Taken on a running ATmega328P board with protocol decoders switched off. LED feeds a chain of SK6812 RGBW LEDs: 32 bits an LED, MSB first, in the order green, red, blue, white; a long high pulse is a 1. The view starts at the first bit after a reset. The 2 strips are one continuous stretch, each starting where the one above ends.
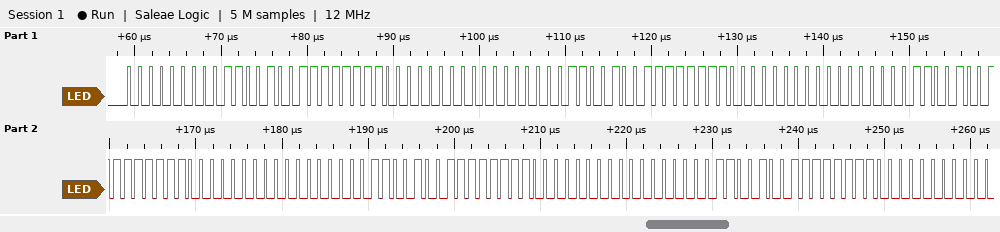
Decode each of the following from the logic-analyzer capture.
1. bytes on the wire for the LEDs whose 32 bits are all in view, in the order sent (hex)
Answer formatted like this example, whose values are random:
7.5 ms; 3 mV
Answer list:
00 64 FF 00 00 64 FF 00 00 64 FF 00 00 64 FF 00 00 64 FF 00
